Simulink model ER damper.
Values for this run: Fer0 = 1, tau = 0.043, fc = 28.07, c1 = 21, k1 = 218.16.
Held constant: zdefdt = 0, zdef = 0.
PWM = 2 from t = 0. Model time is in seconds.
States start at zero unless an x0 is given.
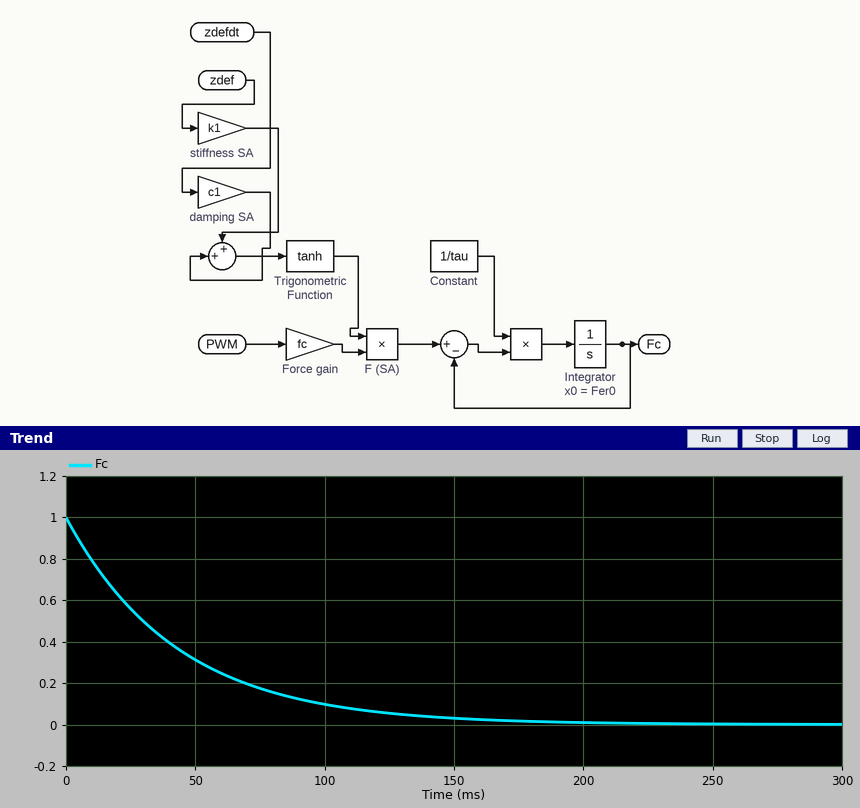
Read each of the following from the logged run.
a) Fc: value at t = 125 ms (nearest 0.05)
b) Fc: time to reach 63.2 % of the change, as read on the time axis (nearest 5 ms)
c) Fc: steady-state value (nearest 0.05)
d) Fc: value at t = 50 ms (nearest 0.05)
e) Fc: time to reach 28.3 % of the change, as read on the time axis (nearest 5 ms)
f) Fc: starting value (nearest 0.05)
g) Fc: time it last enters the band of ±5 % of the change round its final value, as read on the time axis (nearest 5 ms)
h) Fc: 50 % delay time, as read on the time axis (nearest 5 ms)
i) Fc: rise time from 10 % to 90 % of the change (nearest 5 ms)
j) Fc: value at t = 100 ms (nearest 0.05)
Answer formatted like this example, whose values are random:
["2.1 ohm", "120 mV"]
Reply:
["0.05", "45 ms", "0.00", "0.30", "15 ms", "1.00", "130 ms", "30 ms", "95 ms", "0.10"]
